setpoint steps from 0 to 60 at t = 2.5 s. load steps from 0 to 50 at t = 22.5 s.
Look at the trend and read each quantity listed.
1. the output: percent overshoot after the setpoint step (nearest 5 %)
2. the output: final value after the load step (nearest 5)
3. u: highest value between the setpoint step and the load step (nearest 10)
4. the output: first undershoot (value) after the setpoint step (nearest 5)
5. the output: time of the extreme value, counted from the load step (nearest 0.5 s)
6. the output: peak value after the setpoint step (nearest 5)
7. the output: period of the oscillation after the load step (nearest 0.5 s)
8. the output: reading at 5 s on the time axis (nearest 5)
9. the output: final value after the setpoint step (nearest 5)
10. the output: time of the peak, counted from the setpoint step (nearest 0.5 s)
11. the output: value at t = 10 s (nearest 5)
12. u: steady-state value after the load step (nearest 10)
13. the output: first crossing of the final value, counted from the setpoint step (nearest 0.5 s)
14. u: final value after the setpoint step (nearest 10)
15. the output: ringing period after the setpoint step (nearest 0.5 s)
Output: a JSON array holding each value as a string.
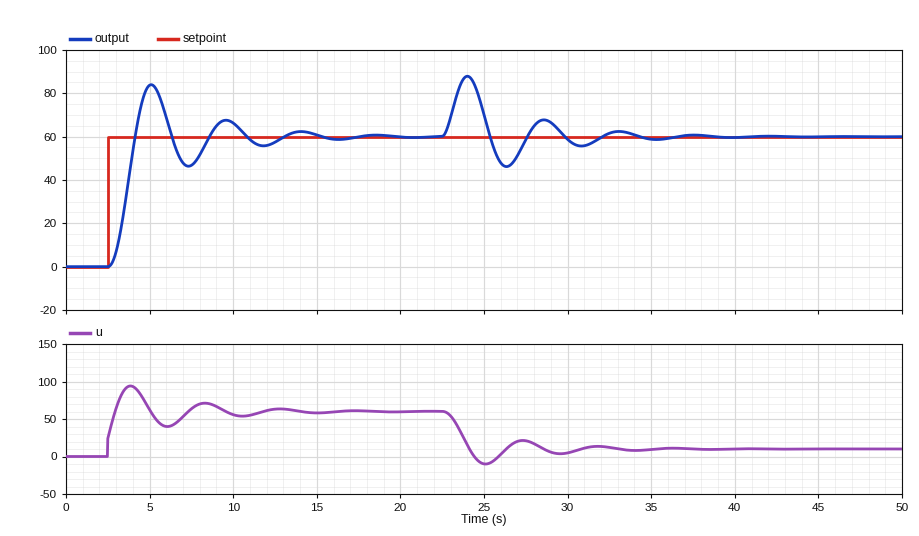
["40 %", "60", "90", "45", "1.5 s", "85", "4.5 s", "85", "60", "2.5 s", "65", "10", "1.5 s", "60", "4.5 s"]
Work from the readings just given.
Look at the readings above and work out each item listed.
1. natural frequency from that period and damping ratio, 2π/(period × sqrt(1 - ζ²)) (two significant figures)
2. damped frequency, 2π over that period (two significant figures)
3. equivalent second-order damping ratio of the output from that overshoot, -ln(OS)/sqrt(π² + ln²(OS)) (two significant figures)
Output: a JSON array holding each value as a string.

["1.5 rad/s", "1.4 rad/s", "0.28"]
